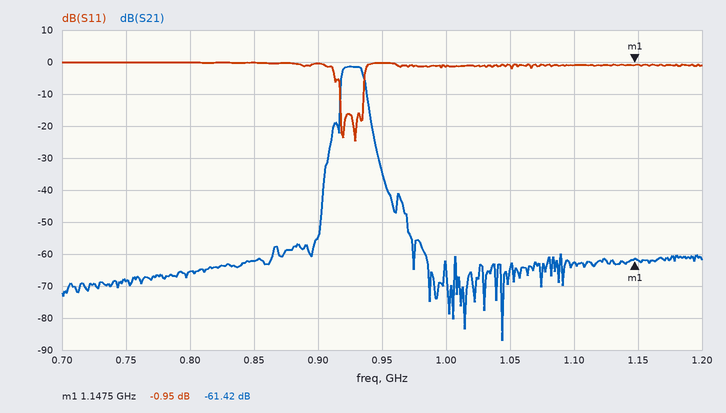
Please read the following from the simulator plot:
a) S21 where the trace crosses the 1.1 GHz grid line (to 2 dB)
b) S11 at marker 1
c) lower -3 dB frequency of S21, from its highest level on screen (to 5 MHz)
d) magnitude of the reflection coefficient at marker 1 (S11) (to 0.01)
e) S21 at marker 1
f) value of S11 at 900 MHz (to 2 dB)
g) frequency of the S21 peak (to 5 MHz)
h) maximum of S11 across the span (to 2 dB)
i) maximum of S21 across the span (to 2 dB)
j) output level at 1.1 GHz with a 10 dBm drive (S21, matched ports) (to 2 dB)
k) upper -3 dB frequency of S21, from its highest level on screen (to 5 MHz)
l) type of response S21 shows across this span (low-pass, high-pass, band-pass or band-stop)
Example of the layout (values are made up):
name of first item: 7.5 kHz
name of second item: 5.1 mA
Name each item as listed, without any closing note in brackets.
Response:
S21 where the trace crosses the 1.1 GHz grid line: -62 dB
S11 at marker 1: -0.95 dB
lower -3 dB frequency of S21, from its highest level on screen: 920 MHz
magnitude of the reflection coefficient at marker 1 (S11): 0.90
S21 at marker 1: -61.42 dB
value of S11 at 900 MHz: 0 dB
frequency of the S21 peak: 925 MHz
maximum of S11 across the span: 0 dB
maximum of S21 across the span: -2 dB
output level at 1.1 GHz with a 10 dBm drive (S21, matched ports): -52 dBm
upper -3 dB frequency of S21, from its highest level on screen: 935 MHz
type of response S21 shows across this span: band-pass
